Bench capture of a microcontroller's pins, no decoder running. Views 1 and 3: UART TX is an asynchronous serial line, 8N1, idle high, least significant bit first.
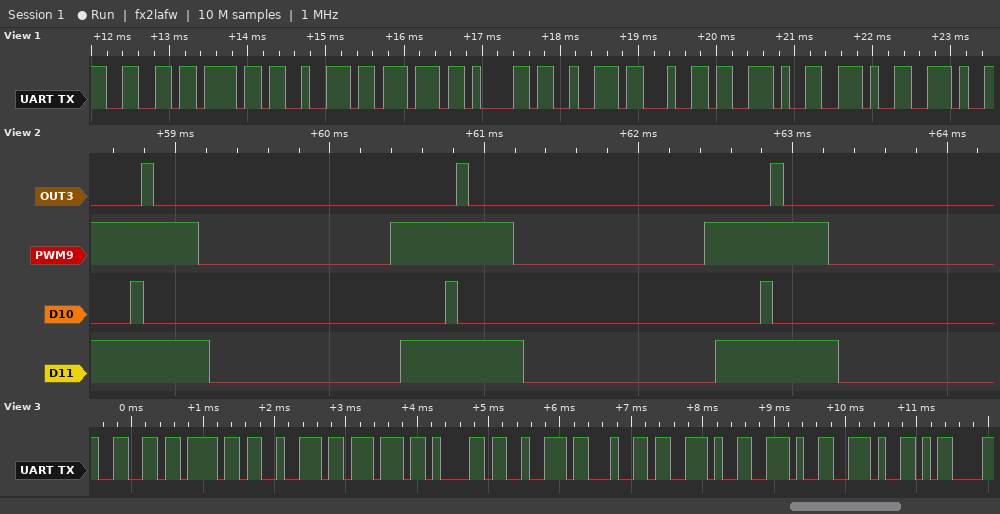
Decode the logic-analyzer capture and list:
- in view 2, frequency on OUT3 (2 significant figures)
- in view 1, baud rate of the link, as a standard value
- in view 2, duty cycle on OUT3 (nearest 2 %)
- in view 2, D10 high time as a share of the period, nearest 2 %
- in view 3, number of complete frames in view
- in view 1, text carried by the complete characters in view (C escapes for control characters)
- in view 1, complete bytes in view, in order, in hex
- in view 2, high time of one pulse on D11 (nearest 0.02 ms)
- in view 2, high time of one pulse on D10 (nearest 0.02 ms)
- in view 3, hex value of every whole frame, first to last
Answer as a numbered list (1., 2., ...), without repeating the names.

1. 490 Hz
2. 9600 baud
3. 4 %
4. 4 %
5. 11
6. "forward..."
7. 66 6F 72 77 61 72 64 2E 2E 2E
8. 0.80 ms
9. 0.08 ms
10. 66 6F 72 77 61 72 64 2E 2E 2E 0D
